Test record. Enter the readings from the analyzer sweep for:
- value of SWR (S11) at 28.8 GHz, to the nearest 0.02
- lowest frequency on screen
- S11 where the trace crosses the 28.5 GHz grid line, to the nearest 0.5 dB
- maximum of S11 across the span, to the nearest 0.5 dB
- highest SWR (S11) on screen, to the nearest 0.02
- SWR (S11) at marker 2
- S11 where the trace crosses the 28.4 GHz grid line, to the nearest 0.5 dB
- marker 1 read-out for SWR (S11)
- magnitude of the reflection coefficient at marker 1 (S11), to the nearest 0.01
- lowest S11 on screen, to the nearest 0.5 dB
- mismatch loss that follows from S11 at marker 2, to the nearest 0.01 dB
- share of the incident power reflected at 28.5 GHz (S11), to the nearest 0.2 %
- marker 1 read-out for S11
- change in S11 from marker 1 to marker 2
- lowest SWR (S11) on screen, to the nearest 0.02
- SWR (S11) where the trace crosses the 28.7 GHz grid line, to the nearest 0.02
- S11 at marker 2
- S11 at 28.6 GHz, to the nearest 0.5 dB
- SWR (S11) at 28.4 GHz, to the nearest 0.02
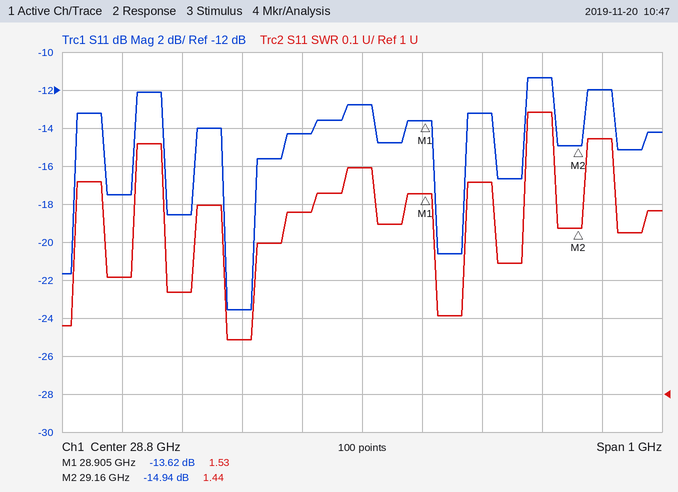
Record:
1.60
28.3 GHz
-18.5 dB
-11.5 dB
1.74
1.44
-17.5 dB
1.53
0.21
-23.5 dB
0.14 dB
1.4 %
-13.62 dB
-1.32 dB
1.14
1.48
-14.94 dB
-23.5 dB
1.30
